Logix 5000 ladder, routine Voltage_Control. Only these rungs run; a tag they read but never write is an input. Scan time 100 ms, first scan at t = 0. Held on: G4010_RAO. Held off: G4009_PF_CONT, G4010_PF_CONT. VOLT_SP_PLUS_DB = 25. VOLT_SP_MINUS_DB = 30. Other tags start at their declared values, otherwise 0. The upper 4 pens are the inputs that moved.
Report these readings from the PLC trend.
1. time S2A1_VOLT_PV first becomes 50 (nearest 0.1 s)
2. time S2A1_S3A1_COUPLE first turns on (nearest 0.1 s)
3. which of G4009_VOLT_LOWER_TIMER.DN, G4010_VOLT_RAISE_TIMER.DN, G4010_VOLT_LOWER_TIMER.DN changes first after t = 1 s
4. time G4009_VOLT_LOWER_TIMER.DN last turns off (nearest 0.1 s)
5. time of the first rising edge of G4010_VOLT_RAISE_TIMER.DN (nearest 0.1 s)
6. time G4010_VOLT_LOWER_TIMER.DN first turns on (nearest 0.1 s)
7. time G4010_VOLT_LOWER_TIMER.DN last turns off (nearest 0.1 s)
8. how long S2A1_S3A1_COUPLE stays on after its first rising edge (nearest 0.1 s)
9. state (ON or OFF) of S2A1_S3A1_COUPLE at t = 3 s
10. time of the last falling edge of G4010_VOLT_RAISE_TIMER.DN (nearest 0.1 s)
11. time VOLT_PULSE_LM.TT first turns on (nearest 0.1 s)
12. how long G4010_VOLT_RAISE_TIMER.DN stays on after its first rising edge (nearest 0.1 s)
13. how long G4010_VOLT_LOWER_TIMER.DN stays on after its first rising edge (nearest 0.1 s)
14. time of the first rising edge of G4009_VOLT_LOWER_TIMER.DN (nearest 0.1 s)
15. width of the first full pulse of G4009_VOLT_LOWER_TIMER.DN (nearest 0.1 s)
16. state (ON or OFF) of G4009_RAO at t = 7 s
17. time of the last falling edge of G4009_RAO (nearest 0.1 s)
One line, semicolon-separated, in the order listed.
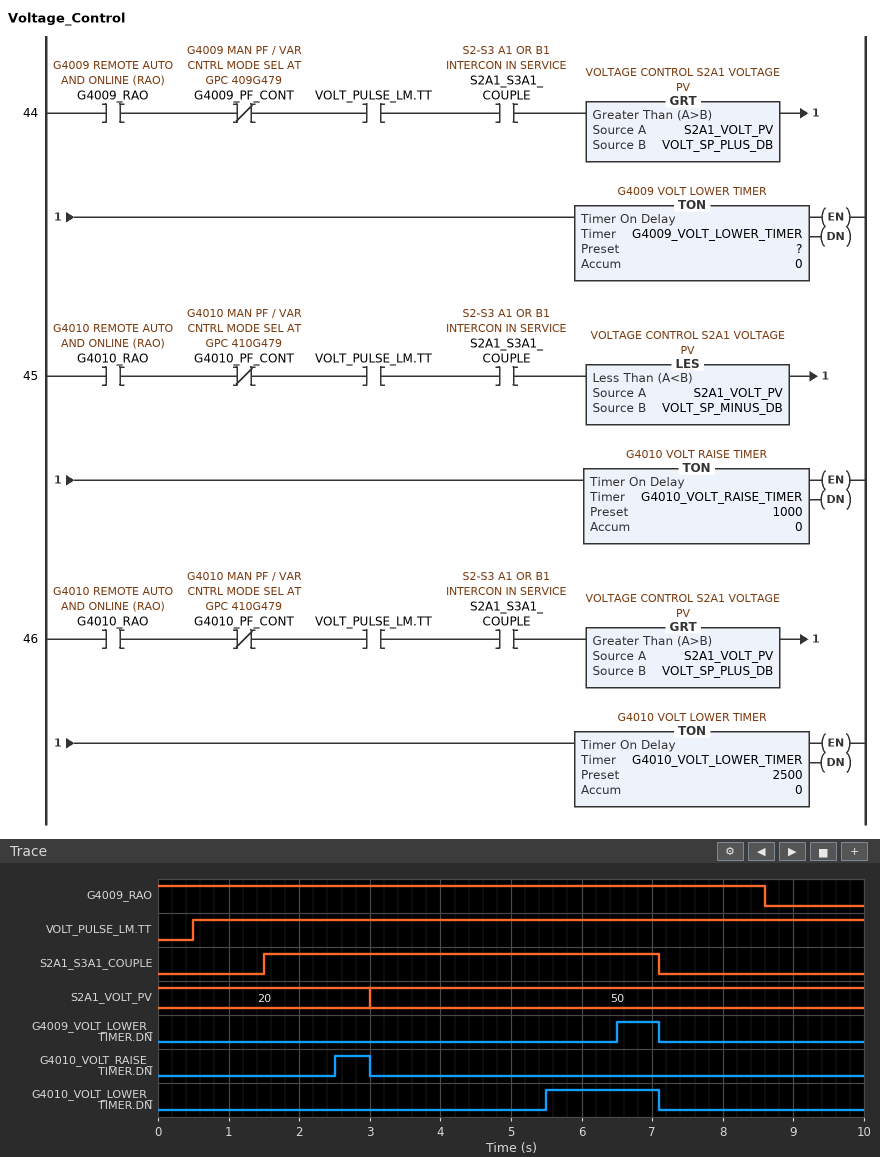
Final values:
3.0 s; 1.5 s; G4010_VOLT_RAISE_TIMER.DN; 7.1 s; 2.5 s; 5.5 s; 7.1 s; 5.6 s; ON; 3.0 s; 0.5 s; 0.5 s; 1.6 s; 6.5 s; 0.6 s; ON; 8.6 s
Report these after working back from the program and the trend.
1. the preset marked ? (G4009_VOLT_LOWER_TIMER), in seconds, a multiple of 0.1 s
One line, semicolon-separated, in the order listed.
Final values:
3.5 s
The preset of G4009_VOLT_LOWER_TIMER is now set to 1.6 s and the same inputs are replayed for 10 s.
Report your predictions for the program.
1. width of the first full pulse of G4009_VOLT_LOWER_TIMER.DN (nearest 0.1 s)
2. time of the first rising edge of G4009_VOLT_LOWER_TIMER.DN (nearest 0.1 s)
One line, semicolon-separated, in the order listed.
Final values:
2.5 s; 4.6 s
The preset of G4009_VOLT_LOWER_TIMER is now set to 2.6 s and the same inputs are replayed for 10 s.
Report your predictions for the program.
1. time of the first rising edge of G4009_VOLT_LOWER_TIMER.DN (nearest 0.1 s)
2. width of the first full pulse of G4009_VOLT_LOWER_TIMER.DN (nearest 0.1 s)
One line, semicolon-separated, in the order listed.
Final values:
5.6 s; 1.5 s
